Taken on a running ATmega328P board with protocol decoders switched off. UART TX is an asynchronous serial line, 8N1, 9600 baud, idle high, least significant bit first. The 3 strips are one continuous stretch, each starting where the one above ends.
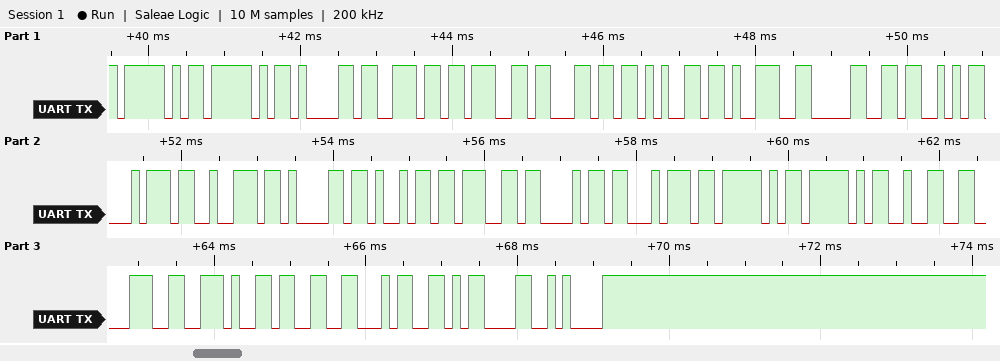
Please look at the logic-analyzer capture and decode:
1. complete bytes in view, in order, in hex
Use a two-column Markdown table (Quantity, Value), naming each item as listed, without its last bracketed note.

| Quantity | Value |
|---|---|
| complete bytes in view, in order, in hex | 5F 5F 61 6E 67 6C 65 39 30 53 74 72 61 69 67 68 74 5F 5F 32 38 2E 33 34 0D 0A |
